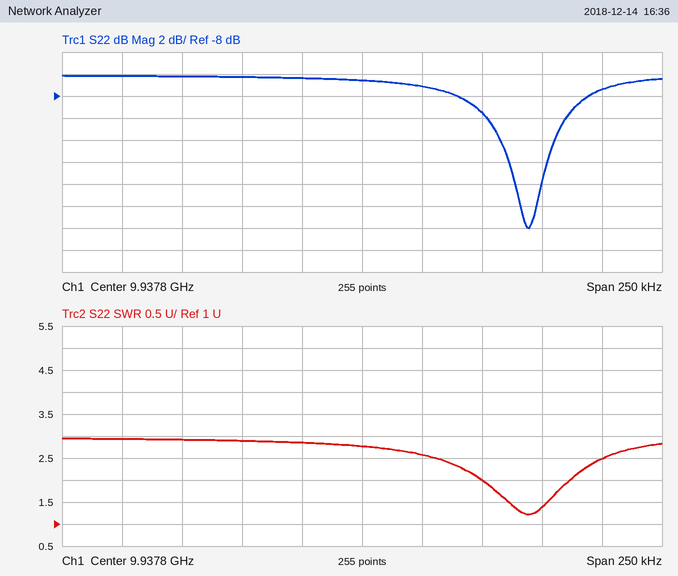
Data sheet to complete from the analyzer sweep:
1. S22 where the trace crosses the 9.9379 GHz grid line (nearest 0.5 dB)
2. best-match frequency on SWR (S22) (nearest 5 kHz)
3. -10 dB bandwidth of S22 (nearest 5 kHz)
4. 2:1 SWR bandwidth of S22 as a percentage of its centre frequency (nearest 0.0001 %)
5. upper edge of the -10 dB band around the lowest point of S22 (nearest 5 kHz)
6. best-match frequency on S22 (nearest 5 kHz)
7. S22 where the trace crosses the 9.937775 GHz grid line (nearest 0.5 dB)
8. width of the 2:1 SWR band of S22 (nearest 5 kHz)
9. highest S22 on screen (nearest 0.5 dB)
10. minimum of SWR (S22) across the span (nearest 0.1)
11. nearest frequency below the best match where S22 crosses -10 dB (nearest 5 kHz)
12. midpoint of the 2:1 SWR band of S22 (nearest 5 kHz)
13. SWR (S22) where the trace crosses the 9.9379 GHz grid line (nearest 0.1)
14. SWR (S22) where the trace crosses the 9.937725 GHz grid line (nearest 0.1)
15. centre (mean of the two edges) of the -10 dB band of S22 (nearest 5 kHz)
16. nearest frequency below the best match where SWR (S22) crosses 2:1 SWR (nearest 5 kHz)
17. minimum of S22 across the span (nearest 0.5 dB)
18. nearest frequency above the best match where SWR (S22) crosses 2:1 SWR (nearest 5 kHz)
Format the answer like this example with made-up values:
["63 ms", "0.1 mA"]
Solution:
["-7.5 dB", "9.937870 GHz", "35 kHz", "0.0004 %", "9.937885 GHz", "9.937870 GHz", "-6.5 dB", "35 kHz", "-6.0 dB", "1.2", "9.937850 GHz", "9.937870 GHz", "2.5", "2.9", "9.937870 GHz", "9.937850 GHz", "-20.0 dB", "9.937885 GHz"]
